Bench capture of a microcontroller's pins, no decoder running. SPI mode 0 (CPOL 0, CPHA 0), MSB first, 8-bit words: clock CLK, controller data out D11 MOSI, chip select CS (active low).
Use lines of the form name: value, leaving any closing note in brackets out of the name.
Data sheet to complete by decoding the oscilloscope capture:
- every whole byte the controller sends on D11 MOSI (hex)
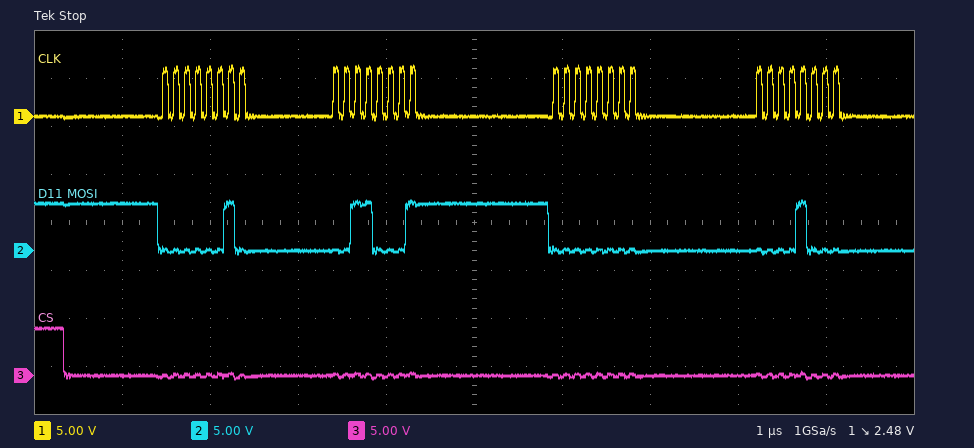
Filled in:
every whole byte the controller sends on D11 MOSI: 02 31 00 08
